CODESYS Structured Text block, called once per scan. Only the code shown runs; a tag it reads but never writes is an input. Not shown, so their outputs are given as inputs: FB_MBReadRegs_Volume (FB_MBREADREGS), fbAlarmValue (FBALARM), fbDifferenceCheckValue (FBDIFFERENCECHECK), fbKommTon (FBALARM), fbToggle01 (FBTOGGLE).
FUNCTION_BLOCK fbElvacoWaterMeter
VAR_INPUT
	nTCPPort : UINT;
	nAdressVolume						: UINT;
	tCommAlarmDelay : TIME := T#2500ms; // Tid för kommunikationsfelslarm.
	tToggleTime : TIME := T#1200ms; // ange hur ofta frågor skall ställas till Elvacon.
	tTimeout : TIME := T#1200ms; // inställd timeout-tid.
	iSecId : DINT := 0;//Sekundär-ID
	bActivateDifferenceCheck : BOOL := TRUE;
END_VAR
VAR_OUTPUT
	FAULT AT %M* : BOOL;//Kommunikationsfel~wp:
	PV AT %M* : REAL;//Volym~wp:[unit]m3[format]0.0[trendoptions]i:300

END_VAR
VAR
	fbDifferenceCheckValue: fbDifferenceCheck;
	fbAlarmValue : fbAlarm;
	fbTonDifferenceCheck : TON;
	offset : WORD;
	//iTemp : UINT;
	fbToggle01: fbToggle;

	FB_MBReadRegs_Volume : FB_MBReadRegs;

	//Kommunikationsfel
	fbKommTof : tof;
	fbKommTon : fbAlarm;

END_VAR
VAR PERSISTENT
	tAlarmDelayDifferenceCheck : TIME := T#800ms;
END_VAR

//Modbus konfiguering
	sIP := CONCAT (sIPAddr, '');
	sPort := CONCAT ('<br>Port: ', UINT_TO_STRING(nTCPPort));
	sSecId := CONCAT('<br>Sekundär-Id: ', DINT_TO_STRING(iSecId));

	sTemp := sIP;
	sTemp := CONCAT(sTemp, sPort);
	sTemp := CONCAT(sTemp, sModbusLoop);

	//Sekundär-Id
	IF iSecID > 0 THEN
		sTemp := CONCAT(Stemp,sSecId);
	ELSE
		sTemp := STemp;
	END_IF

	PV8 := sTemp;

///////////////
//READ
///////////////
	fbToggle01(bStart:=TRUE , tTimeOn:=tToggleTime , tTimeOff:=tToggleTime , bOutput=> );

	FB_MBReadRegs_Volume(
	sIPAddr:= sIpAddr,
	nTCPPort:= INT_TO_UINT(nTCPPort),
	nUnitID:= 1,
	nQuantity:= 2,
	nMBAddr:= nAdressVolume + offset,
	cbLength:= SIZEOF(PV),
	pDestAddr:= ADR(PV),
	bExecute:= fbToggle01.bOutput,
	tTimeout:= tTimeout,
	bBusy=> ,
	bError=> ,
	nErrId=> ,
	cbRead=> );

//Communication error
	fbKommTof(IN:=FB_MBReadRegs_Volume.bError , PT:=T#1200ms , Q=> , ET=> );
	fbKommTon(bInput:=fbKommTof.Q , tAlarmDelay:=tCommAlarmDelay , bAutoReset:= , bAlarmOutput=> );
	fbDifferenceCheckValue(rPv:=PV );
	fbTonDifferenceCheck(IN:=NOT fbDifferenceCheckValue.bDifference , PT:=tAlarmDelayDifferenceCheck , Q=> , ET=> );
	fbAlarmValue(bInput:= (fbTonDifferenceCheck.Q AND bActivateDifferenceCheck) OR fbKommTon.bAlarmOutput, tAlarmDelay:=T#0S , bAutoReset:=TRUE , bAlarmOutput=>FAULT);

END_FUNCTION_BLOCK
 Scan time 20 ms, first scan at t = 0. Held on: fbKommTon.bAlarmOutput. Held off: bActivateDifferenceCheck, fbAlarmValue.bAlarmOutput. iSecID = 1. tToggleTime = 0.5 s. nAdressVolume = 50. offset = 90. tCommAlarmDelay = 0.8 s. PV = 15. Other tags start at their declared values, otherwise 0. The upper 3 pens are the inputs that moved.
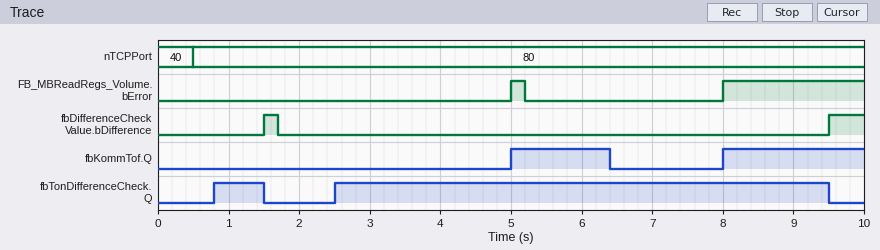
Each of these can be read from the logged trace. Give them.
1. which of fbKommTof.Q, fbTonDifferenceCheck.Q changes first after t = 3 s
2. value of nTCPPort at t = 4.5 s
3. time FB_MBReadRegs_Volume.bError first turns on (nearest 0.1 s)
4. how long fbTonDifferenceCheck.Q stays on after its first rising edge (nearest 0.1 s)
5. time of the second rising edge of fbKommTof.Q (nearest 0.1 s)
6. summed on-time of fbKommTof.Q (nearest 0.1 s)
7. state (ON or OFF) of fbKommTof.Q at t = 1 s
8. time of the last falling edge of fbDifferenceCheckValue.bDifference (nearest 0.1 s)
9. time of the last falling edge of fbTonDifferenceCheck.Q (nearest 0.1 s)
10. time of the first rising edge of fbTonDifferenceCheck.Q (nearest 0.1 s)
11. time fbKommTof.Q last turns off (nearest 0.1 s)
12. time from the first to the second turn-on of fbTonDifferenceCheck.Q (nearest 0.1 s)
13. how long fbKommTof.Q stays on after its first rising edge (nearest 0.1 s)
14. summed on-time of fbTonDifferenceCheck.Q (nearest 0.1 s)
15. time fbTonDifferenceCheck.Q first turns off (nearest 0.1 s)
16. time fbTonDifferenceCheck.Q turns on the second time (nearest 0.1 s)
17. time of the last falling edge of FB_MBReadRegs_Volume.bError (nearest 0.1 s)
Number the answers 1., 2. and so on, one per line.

1. fbKommTof.Q
2. 80
3. 5.0 s
4. 0.7 s
5. 8.0 s
6. 3.4 s
7. OFF
8. 1.7 s
9. 9.5 s
10. 0.8 s
11. 6.4 s
12. 1.7 s
13. 1.4 s
14. 7.7 s
15. 1.5 s
16. 2.5 s
17. 5.2 s
